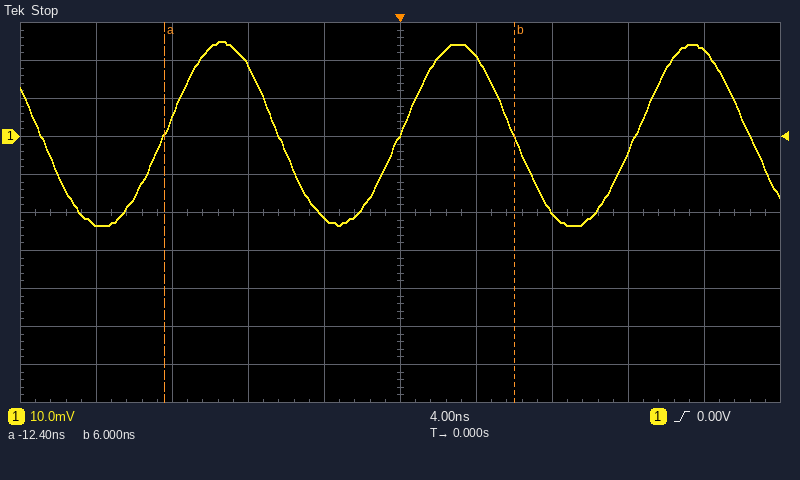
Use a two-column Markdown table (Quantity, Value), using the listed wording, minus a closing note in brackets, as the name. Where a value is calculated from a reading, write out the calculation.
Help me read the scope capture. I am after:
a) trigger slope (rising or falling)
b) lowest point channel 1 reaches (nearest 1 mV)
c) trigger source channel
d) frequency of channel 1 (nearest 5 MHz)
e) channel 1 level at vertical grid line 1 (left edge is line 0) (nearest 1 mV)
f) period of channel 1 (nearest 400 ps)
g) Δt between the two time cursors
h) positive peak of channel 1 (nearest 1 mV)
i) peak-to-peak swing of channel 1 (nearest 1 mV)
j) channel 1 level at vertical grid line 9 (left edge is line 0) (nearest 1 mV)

| Quantity | Value |
|---|---|
| trigger slope | rising |
| lowest point channel 1 reaches | -23 mV |
| trigger source channel | channel 1 |
| frequency of channel 1 | 1 / 12.4 ns ≈ 80.6 MHz, so 80 MHz to the nearest 5 MHz |
| channel 1 level at vertical grid line 1 (left edge is line 0) | -23 mV |
| period of channel 1 | 12.4 ns |
| Δt between the two time cursors | 6 ns − (-12.4 ns) = 18.4 ns |
| positive peak of channel 1 | 25 mV |
| peak-to-peak swing of channel 1 | 25 mV − (-23 mV) = 48 mV |
| channel 1 level at vertical grid line 9 (left edge is line 0) | 23 mV |
